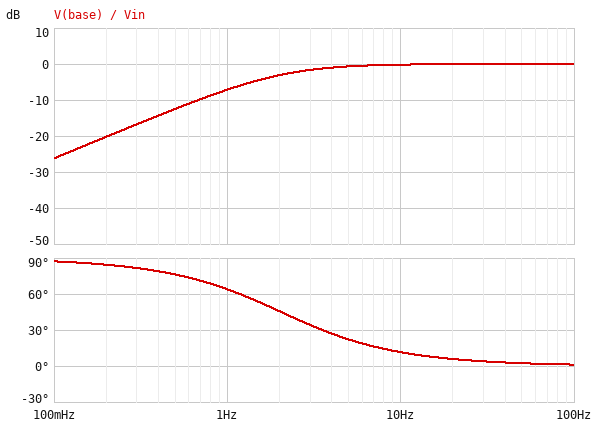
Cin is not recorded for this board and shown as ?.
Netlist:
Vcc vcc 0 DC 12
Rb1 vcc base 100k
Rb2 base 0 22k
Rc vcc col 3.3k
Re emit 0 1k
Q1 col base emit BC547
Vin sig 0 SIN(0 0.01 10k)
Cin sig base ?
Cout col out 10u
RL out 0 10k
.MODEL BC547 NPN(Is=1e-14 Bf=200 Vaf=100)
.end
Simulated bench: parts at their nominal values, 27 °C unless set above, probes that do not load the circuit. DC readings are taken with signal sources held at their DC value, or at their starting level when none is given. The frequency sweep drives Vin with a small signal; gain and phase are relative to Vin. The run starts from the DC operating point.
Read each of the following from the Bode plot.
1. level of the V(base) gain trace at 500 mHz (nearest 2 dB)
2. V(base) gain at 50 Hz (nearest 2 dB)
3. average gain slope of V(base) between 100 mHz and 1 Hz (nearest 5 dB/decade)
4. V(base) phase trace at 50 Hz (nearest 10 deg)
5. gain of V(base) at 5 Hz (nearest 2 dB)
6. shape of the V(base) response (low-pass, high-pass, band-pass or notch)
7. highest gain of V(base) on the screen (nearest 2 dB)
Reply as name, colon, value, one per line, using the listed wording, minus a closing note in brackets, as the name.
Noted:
level of the V(base) gain trace at 500 mHz: -12 dB
V(base) gain at 50 Hz: 0 dB
average gain slope of V(base) between 100 mHz and 1 Hz: 20 dB/decade
V(base) phase trace at 50 Hz: 0 deg
gain of V(base) at 5 Hz: 0 dB
shape of the V(base) response: high-pass
highest gain of V(base) on the screen: 0 dB
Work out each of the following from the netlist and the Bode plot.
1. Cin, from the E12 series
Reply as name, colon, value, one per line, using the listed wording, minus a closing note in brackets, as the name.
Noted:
Cin, from the E12 series: 4.7 µF
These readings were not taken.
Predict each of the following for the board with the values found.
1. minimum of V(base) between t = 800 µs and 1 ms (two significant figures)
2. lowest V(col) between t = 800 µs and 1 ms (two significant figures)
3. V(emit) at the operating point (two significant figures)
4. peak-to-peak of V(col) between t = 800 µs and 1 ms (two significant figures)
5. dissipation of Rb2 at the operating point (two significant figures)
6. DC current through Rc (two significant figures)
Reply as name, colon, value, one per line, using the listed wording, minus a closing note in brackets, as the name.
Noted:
minimum of V(base) between t = 800 µs and 1 ms: 2.0 V
lowest V(col) between t = 800 µs and 1 ms: 7.4 V
V(emit) at the operating point: 1.4 V
peak-to-peak of V(col) between t = 800 µs and 1 ms: 48 mV
dissipation of Rb2 at the operating point: 190 µW
DC current through Rc: 1.4 mA
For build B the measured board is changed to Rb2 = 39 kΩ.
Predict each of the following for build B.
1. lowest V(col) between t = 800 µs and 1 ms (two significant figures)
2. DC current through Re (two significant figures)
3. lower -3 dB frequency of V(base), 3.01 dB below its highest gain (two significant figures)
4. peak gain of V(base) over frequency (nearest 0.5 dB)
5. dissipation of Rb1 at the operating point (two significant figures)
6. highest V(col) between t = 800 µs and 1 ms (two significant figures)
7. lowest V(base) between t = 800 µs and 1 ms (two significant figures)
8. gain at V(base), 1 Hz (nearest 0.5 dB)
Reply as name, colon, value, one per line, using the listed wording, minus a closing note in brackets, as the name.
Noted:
lowest V(col) between t = 800 µs and 1 ms: 4.2 V
DC current through Re: 2.4 mA
lower -3 dB frequency of V(base), 3.01 dB below its highest gain: 1.4 Hz
peak gain of V(base) over frequency: 0 dB
dissipation of Rb1 at the operating point: 800 µW
highest V(col) between t = 800 µs and 1 ms: 4.3 V
lowest V(base) between t = 800 µs and 1 ms: 3.0 V
gain at V(base), 1 Hz: -4.5 dB
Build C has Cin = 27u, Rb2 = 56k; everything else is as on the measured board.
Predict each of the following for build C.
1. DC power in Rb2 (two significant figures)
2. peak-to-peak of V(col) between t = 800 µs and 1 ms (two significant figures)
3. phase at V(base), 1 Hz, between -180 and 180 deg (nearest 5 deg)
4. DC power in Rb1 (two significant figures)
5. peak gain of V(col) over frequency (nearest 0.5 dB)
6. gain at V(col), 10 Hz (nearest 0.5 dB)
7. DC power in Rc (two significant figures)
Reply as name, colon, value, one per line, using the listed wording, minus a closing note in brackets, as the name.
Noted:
DC power in Rb2: 210 µW
peak-to-peak of V(col) between t = 800 µs and 1 ms: 16 mV
phase at V(base), 1 Hz, between -180 and 180 deg: 80 deg
DC power in Rb1: 730 µW
peak gain of V(col) over frequency: -2.5 dB
gain at V(col), 10 Hz: -3.0 dB
DC power in Rc: 25 mW
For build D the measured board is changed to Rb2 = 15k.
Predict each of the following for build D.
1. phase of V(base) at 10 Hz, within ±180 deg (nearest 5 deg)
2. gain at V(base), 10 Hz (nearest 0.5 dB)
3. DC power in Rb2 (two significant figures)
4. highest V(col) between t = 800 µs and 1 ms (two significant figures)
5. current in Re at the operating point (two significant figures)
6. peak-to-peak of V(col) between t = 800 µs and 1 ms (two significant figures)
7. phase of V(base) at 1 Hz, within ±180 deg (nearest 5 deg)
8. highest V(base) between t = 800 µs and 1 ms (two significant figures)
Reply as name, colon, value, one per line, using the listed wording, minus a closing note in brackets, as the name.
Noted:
phase of V(base) at 10 Hz, within ±180 deg: 15 deg
gain at V(base), 10 Hz: -0.5 dB
DC power in Rb2: 150 µW
highest V(col) between t = 800 µs and 1 ms: 9.2 V
current in Re at the operating point: 860 µA
peak-to-peak of V(col) between t = 800 µs and 1 ms: 48 mV
phase of V(base) at 1 Hz, within ±180 deg: 70 deg
highest V(base) between t = 800 µs and 1 ms: 1.5 V
